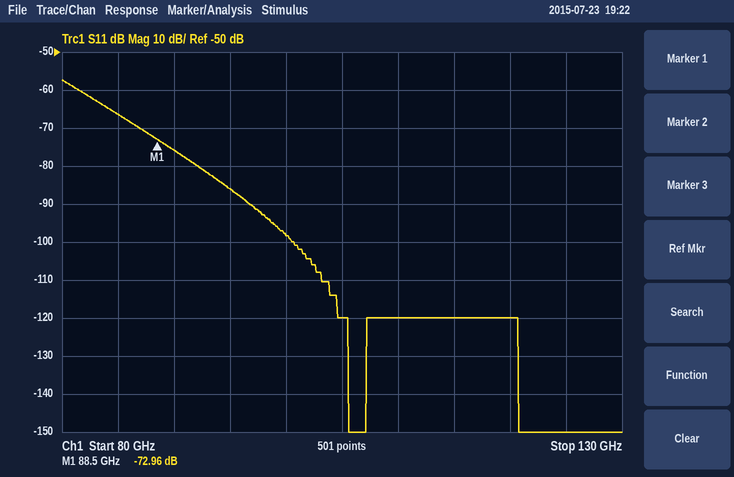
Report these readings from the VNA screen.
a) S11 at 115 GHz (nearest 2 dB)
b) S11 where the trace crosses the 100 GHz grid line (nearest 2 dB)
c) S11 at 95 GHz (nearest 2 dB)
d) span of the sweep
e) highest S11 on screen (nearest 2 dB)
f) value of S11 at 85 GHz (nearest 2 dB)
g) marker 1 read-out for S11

-120 dB
-98 dB
-86 dB
50 GHz
-58 dB
-66 dB
-72.96 dB
